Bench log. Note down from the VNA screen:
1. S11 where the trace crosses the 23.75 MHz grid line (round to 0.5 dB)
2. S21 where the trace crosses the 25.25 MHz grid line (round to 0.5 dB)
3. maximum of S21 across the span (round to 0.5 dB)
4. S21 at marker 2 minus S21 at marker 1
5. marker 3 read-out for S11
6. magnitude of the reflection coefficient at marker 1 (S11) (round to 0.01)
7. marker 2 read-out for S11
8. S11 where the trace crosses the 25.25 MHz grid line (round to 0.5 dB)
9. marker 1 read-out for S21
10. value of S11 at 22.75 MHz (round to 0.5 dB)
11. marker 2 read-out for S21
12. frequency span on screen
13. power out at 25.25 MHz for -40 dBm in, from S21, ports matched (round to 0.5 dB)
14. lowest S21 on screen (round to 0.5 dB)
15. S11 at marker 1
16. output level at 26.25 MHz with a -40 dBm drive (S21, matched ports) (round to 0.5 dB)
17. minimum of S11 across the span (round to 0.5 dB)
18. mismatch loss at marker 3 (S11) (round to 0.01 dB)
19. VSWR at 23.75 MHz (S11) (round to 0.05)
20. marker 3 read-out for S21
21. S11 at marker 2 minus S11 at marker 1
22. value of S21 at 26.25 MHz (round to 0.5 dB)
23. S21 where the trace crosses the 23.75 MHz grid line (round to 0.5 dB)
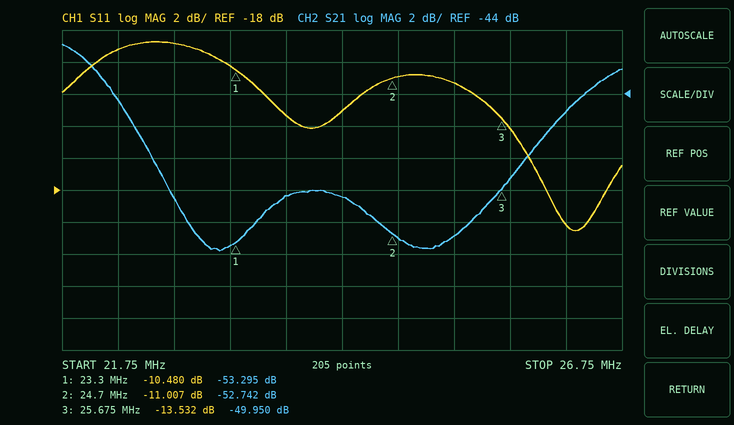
-13.5 dB
-53.0 dB
-41.0 dB
0.553 dB
-13.532 dB
0.30
-11.007 dB
-11.5 dB
-53.295 dB
-9.0 dB
-52.742 dB
5 MHz
-93.0 dBm
-54.0 dB
-10.480 dB
-85.0 dBm
-20.5 dB
0.20 dB
1.55
-49.950 dB
-0.527 dB
-45.0 dB
-50.5 dB
